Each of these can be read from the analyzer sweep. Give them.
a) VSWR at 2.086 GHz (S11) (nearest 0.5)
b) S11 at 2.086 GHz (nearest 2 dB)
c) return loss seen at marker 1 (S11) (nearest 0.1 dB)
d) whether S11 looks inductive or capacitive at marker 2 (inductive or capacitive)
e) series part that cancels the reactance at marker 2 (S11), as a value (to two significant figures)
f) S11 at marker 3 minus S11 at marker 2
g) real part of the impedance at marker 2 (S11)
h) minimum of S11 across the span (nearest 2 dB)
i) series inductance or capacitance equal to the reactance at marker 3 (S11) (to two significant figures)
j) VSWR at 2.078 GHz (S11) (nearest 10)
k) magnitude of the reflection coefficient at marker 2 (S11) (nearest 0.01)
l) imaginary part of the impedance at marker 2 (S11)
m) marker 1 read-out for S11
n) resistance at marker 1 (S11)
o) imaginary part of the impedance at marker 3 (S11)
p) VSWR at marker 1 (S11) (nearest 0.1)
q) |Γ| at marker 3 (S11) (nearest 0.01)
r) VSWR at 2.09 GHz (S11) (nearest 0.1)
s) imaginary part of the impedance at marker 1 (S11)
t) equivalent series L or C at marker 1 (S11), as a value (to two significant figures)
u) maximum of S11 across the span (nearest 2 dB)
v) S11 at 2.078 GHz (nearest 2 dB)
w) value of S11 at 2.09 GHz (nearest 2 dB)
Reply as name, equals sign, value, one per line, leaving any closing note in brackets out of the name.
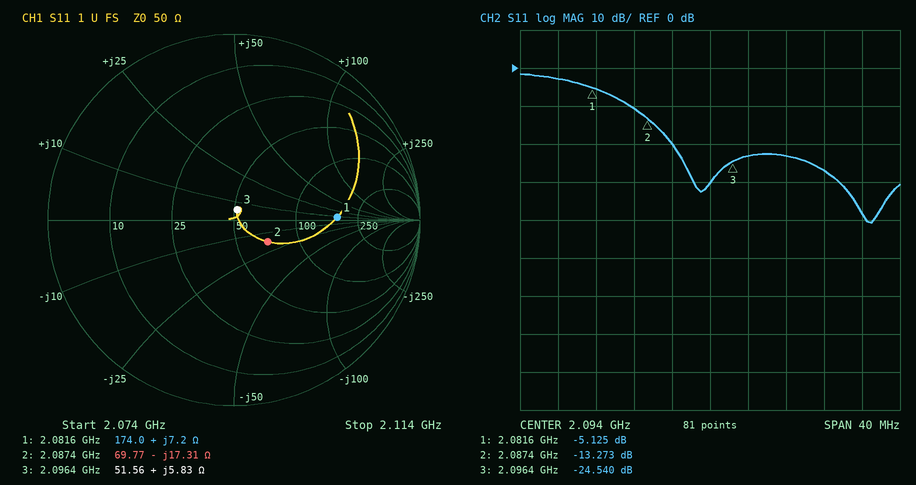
VSWR at 2.086 GHz (S11) = 2.0
S11 at 2.086 GHz = -10 dB
return loss seen at marker 1 (S11) = 5.1 dB
whether S11 looks inductive or capacitive at marker 2 = capacitive
series part that cancels the reactance at marker 2 (S11), as a value = 1.3 nH
S11 at marker 3 minus S11 at marker 2 = -11.267 dB
real part of the impedance at marker 2 = 69.77 Ω
minimum of S11 across the span = -40 dB
series inductance or capacitance equal to the reactance at marker 3 (S11) = 440 pH
VSWR at 2.078 GHz (S11) = 10
magnitude of the reflection coefficient at marker 2 (S11) = 0.22
imaginary part of the impedance at marker 2 = -17.31 Ω
marker 1 read-out for S11 = -5.125 dB
resistance at marker 1 = 174.0 Ω
imaginary part of the impedance at marker 3 = +5.83 Ω
VSWR at marker 1 (S11) = 3.5
|Γ| at marker 3 (S11) = 0.06
VSWR at 2.09 GHz (S11) = 1.2
imaginary part of the impedance at marker 1 = +7.2 Ω
equivalent series L or C at marker 1 (S11), as a value = 550 pH
maximum of S11 across the span = -2 dB
S11 at 2.078 GHz = -2 dB
value of S11 at 2.09 GHz = -20 dB
